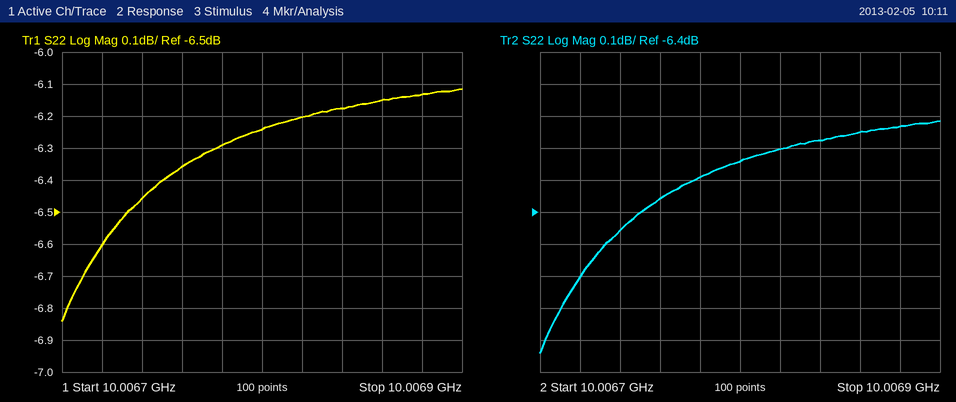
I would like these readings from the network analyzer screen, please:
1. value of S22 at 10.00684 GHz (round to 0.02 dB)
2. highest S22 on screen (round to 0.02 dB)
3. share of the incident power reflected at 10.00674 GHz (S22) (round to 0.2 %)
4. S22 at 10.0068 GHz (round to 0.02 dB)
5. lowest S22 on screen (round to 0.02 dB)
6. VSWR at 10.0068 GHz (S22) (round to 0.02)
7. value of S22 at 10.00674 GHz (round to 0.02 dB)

-6.18 dB
-6.12 dB
22.6 %
-6.24 dB
-6.84 dB
2.90
-6.46 dB
